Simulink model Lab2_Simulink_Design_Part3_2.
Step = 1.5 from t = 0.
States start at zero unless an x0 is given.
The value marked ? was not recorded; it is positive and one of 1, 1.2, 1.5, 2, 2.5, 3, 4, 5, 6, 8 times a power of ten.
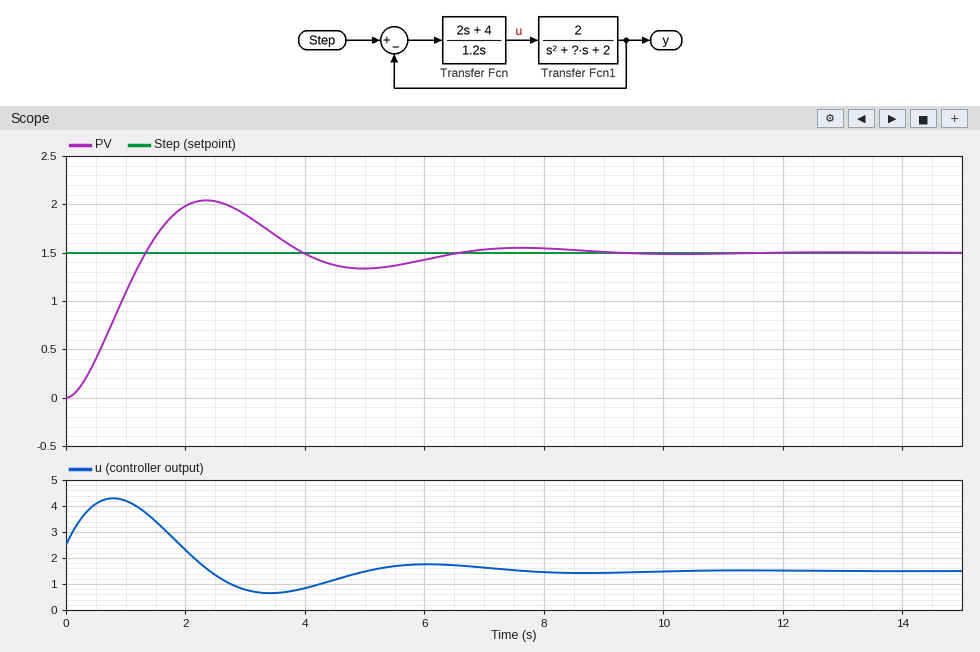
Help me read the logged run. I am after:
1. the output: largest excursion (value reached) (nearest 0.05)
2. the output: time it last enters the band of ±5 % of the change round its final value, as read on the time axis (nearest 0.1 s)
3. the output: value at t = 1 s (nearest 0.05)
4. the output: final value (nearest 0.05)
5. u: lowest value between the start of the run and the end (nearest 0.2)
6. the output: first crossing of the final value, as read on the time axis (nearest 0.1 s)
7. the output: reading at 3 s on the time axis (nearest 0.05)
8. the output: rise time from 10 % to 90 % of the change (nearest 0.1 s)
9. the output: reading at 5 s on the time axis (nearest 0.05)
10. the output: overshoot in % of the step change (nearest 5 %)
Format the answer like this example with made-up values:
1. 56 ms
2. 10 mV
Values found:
1. 2.05
2. 6.0 s
3. 1.10
4. 1.50
5. 0.6
6. 1.3 s
7. 1.90
8. 0.9 s
9. 1.35
10. 35 %
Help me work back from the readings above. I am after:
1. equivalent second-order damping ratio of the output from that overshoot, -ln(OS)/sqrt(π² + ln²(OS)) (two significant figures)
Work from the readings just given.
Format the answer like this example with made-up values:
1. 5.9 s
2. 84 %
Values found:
1. 0.32
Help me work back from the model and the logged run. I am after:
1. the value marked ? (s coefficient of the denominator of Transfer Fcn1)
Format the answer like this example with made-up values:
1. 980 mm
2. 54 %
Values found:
1. 5
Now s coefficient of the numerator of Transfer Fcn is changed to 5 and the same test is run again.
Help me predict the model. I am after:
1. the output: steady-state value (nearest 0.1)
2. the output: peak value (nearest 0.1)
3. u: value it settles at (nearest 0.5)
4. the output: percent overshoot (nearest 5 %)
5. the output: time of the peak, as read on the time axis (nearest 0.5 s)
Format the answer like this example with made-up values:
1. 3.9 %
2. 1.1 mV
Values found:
1. 1.5
2. 1.7
3. 1.5
4. 15 %
5. 1.5 s
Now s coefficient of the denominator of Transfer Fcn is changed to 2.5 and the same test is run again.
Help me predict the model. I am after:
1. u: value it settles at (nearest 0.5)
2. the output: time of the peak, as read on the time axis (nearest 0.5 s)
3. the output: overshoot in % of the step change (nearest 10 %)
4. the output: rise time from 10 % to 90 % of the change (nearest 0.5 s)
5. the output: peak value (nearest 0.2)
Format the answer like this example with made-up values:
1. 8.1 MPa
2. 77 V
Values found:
1. 1.5
2. 3.5 s
3. 30 %
4. 1.5 s
5. 2.0
